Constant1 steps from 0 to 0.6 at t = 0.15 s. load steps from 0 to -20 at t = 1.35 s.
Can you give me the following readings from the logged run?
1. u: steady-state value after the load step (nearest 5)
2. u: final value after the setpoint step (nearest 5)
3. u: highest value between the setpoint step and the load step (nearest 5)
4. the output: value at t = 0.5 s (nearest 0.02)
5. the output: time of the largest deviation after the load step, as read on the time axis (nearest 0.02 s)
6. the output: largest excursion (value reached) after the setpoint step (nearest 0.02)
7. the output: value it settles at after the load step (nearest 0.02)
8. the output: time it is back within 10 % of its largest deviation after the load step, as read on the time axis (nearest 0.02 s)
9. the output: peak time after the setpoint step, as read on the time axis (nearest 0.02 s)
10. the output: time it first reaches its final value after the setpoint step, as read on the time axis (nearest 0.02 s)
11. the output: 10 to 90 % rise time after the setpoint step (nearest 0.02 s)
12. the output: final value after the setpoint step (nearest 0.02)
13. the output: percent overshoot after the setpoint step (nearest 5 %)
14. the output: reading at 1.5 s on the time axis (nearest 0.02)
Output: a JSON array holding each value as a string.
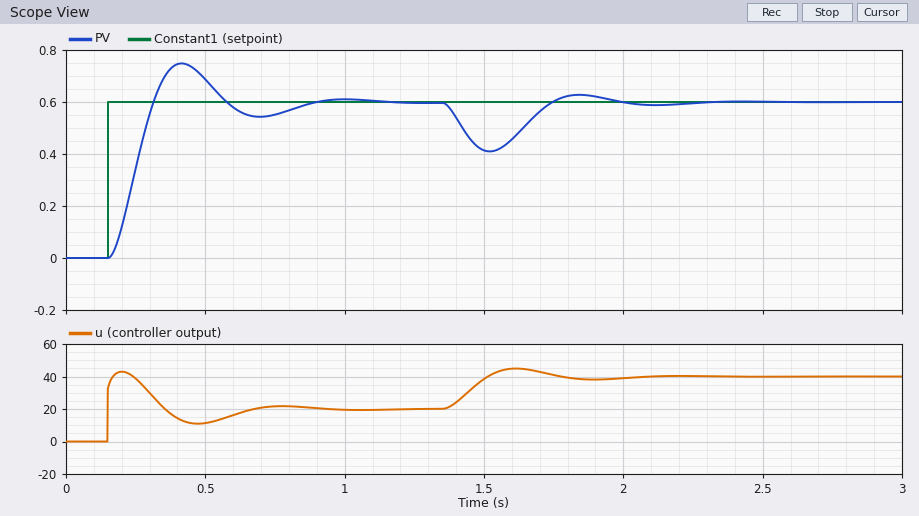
["40", "20", "45", "0.68", "1.52 s", "0.74", "0.60", "1.92 s", "0.42 s", "0.32 s", "0.12 s", "0.60", "25 %", "0.42"]
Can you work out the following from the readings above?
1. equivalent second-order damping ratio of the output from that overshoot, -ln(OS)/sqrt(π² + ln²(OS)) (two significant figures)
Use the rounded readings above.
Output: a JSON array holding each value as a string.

["0.40"]
